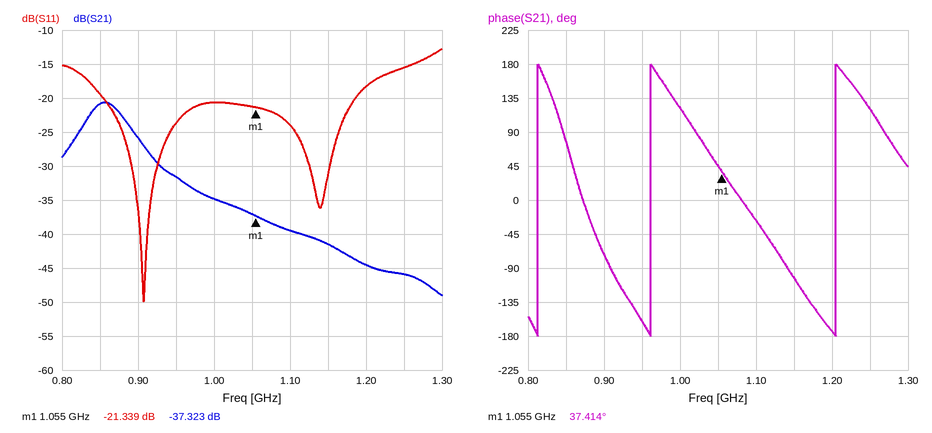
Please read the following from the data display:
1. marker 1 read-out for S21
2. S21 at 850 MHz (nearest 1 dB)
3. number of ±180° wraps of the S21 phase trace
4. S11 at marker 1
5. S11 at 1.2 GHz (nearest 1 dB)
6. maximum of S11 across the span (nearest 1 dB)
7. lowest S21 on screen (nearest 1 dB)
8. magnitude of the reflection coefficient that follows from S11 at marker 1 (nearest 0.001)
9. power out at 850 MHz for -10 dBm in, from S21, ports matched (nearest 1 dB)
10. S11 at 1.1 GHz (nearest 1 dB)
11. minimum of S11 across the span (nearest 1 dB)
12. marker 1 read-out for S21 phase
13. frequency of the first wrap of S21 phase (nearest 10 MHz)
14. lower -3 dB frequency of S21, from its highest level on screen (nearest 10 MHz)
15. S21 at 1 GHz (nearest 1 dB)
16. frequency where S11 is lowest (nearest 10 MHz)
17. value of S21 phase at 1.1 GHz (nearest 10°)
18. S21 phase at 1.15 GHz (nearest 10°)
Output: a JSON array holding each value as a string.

["-37.323 dB", "-21 dB", "3", "-21.339 dB", "-18 dB", "-13 dB", "-49 dB", "0.086", "-31 dBm", "-24 dB", "-50 dB", "37.414°", "810 MHz", "830 MHz", "-35 dB", "910 MHz", "-30°", "-100°"]
